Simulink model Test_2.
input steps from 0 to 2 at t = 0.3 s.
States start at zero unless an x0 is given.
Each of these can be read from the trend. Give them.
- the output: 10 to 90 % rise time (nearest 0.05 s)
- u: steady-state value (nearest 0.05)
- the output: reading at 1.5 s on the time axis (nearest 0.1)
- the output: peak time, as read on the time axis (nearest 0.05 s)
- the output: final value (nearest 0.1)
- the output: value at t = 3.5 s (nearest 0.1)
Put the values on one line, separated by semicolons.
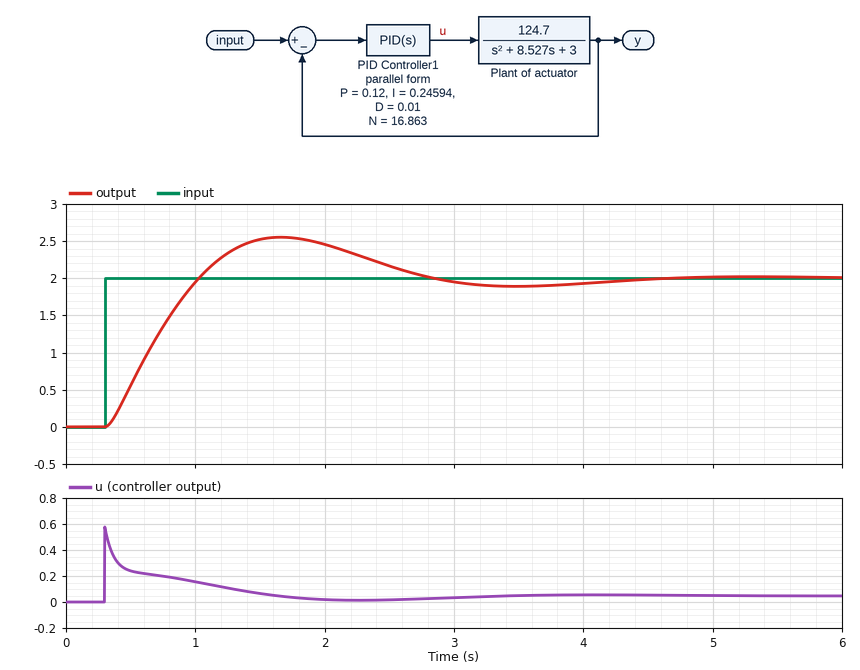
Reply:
0.55 s; 0.05; 2.5; 1.65 s; 2.0; 1.9
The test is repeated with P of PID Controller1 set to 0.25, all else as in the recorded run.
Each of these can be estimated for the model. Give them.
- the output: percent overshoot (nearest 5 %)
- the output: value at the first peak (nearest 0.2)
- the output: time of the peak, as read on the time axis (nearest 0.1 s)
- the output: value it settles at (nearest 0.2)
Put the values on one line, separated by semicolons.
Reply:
10 %; 2.2; 1.2 s; 2.0
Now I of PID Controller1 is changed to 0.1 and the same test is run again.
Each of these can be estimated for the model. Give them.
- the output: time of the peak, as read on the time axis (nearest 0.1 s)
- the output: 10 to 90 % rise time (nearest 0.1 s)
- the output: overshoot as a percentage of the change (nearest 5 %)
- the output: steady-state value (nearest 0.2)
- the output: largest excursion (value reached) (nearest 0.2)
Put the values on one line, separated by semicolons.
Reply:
2.3 s; 0.8 s; 10 %; 2.0; 2.2
